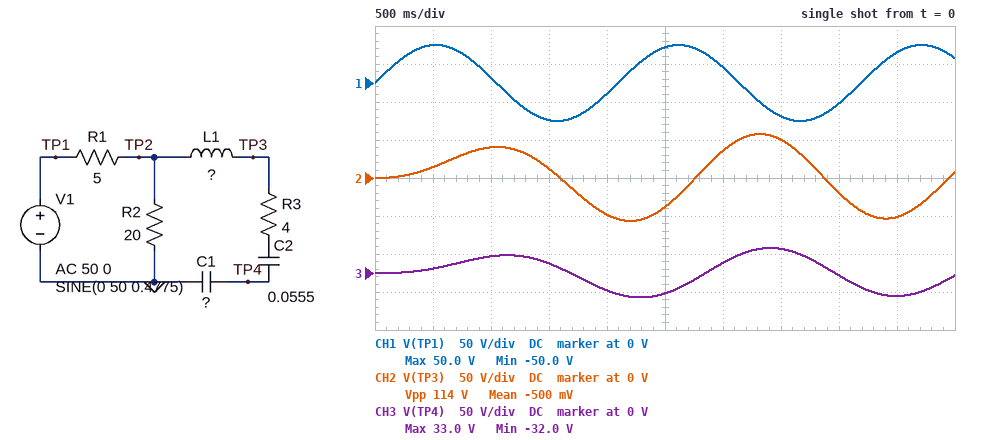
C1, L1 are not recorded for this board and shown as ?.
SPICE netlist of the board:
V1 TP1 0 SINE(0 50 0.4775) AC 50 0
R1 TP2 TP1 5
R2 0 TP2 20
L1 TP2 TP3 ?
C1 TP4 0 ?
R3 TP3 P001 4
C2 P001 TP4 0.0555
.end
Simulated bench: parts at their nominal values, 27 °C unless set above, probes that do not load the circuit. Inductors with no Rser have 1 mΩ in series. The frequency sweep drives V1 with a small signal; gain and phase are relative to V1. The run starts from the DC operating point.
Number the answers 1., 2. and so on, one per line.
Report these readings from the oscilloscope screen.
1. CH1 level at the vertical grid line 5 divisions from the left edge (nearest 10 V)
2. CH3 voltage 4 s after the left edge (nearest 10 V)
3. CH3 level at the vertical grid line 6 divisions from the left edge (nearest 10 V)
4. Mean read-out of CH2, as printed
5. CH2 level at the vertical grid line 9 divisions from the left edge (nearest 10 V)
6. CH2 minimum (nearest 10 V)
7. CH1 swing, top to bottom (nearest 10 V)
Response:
1. 50 V
2. 0 V
3. 10 V
4. -500 mV
5. -50 V
6. -60 V
7. 100 V
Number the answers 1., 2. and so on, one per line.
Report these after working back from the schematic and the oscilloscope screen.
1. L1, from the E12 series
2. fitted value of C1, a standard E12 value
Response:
1. 8.2 H
2. 39 mF
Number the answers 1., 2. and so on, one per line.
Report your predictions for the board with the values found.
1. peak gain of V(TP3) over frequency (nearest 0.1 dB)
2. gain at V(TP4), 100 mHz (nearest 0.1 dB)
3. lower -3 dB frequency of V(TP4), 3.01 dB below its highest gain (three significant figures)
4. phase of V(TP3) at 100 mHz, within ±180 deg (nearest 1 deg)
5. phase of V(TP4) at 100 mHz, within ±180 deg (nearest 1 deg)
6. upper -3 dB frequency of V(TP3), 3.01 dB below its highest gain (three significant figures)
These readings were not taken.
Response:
1. 5.9 dB
2. -6.0 dB
3. 259 mHz
4. -4 deg
5. -7 deg
6. 424 mHz
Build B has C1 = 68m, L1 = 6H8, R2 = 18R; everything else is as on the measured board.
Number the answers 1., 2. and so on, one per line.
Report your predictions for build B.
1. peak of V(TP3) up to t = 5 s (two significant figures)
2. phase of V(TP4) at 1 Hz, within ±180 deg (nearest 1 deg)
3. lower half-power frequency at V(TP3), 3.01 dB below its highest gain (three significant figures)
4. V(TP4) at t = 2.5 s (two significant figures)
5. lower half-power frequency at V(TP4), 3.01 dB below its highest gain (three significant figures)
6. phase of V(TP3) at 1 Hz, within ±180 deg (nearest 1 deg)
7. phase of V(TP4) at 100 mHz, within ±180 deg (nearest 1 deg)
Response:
1. 44 V
2. -168 deg
3. 211 mHz
4. -17 V
5. 206 mHz
6. -131 deg
7. -9 deg
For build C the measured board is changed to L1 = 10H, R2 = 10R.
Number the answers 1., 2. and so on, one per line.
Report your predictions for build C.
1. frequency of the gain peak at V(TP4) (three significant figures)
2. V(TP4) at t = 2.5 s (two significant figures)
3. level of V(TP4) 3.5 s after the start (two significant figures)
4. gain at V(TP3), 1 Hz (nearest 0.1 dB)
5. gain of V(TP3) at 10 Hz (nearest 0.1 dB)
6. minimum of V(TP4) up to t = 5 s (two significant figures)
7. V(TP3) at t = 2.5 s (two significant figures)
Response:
1. 322 mHz
2. -24 V
3. 23 V
4. -20.5 dB
5. -47.3 dB
6. -25 V
7. -37 V
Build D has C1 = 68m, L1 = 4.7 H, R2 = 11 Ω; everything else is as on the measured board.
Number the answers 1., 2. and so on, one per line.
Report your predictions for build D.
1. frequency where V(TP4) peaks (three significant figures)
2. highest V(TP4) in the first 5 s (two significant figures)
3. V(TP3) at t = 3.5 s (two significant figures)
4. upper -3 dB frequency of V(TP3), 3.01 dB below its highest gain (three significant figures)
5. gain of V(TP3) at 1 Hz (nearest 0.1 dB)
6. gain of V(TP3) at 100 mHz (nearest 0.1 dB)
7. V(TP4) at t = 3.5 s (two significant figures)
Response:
1. 380 mHz
2. 21 V
3. 24 V
4. 501 mHz
5. -15.0 dB
6. -2.8 dB
7. 16 V
